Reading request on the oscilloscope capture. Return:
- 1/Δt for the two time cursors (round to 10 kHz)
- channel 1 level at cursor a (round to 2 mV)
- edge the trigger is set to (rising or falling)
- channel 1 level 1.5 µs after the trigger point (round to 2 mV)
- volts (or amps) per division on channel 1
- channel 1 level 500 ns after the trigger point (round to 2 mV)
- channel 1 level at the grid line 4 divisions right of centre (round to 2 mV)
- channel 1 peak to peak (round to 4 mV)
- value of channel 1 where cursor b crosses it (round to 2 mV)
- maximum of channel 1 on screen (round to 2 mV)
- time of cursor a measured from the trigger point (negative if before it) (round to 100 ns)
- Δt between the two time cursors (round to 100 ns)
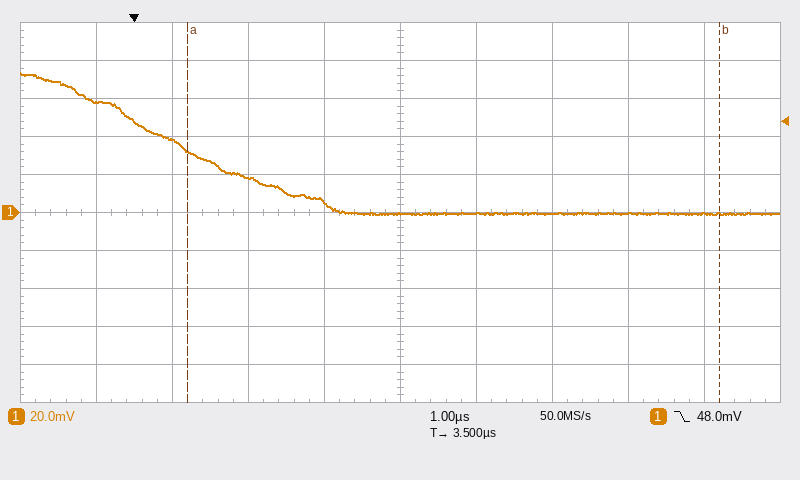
140 kHz
32 mV
falling
18 mV
20 mV
38 mV
0 mV
76 mV
0 mV
74 mV
+700 ns
7.0 µs
